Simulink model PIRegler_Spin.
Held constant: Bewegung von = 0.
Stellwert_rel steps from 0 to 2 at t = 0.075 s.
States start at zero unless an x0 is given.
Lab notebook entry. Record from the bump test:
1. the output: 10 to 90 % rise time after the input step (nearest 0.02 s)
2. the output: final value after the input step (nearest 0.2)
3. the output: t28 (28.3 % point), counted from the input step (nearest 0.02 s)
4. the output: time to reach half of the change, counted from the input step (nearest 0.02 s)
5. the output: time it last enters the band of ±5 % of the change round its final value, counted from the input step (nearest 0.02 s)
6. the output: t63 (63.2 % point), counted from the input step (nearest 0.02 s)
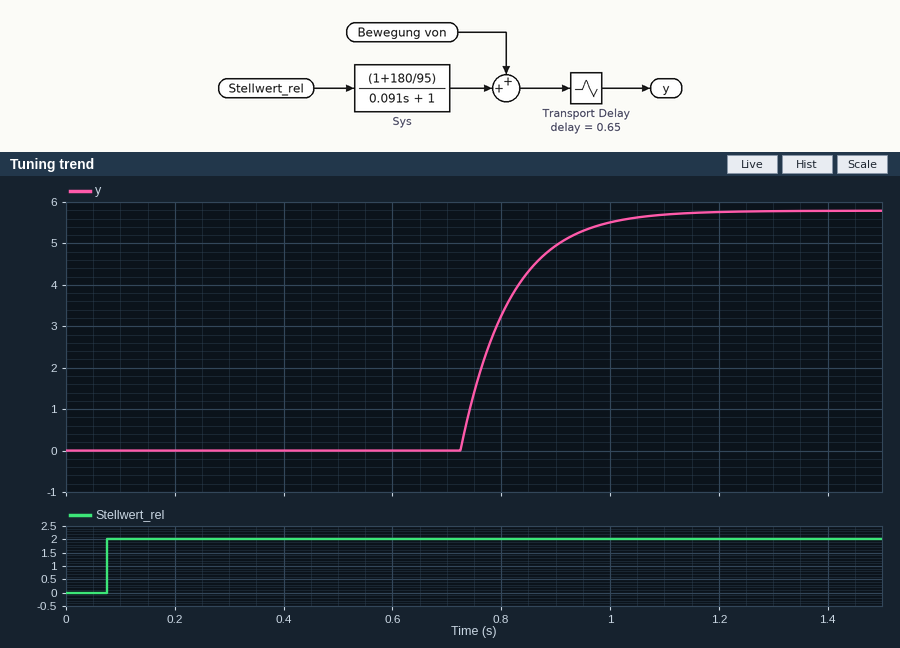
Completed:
0.20 s
5.8
0.68 s
0.72 s
0.92 s
0.74 s
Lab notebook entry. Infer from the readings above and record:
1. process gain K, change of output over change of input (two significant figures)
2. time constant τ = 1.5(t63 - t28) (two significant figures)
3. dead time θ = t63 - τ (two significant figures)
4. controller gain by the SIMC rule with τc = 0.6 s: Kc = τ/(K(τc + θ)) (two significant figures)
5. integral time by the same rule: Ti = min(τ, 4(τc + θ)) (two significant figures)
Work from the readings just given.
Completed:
2.9
0.090 s
0.65 s
0.025
0.090 s
